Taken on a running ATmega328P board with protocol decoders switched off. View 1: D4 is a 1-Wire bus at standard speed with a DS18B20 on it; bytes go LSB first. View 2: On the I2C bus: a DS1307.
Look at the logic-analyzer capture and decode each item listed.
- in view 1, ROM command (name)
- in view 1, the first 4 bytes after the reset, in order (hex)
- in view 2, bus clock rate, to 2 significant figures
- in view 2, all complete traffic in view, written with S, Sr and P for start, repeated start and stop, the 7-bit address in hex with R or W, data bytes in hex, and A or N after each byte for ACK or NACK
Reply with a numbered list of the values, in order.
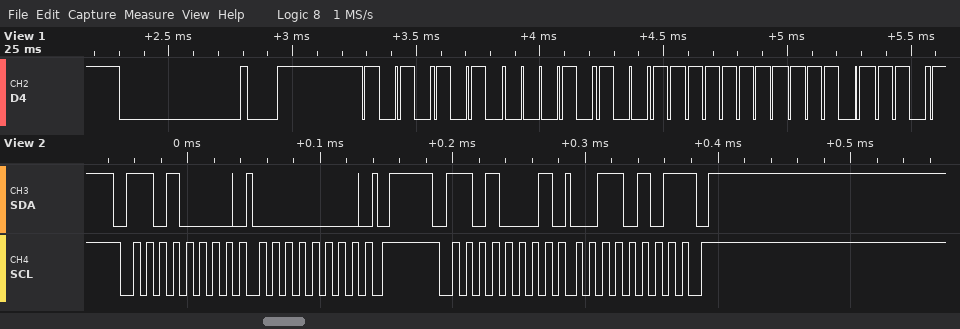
1. Match ROM
2. 55 28 FF 77
3. 100 kHz
4. S 68W A 00 A P S 68R A 35 N P
